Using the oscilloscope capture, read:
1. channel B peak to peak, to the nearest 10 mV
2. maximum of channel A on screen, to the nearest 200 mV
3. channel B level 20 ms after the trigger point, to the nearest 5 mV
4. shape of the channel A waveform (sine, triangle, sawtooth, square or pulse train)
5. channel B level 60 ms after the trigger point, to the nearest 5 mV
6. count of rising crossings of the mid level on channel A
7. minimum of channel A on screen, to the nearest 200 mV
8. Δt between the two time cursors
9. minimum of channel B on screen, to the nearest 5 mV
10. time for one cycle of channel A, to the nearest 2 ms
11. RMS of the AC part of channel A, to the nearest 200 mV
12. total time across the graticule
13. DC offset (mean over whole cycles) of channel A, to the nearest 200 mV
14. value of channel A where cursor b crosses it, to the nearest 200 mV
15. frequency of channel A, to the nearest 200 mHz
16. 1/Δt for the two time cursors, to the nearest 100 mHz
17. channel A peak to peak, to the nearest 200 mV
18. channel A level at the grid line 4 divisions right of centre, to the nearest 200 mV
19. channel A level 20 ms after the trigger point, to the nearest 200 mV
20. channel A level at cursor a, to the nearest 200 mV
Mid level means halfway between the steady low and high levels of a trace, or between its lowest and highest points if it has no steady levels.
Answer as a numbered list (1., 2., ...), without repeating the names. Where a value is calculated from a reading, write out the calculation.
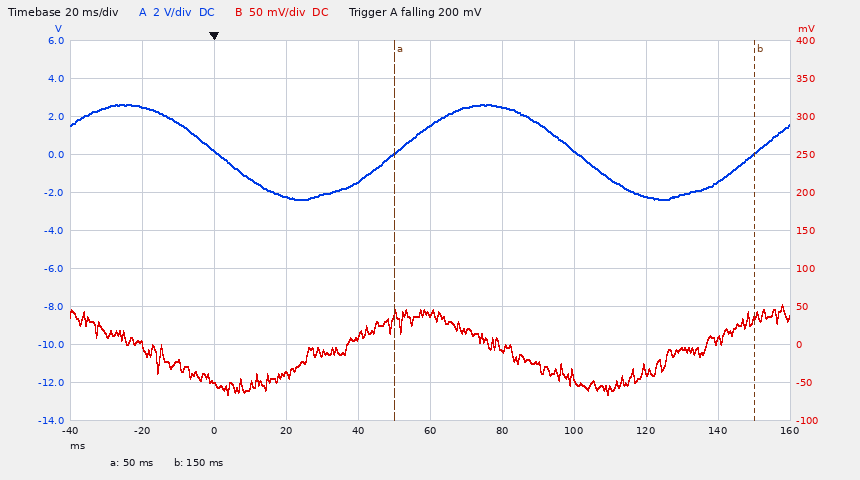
1. 120 mV
2. 2.6 V
3. -40 mV
4. sine
5. 40 mV
6. 2
7. -2.4 V
8. 150 ms − (50 ms) = 100 ms
9. -65 mV
10. 100 ms
11. 5.0 V / (2√2) ≈ 1.8 V
12. 200 ms
13. (2.6 V + (-2.4 V)) / 2 ≈ 100 mV, so 200 mV to the nearest 200 mV
14. 0.0 V
15. 1 / 100 ms ≈ 10.0 Hz
16. 1 / 100 ms ≈ 10.0 Hz
17. 2.6 V − (-2.4 V) = 5.0 V
18. -1.4 V
19. -2.2 V
20. 0.0 V
